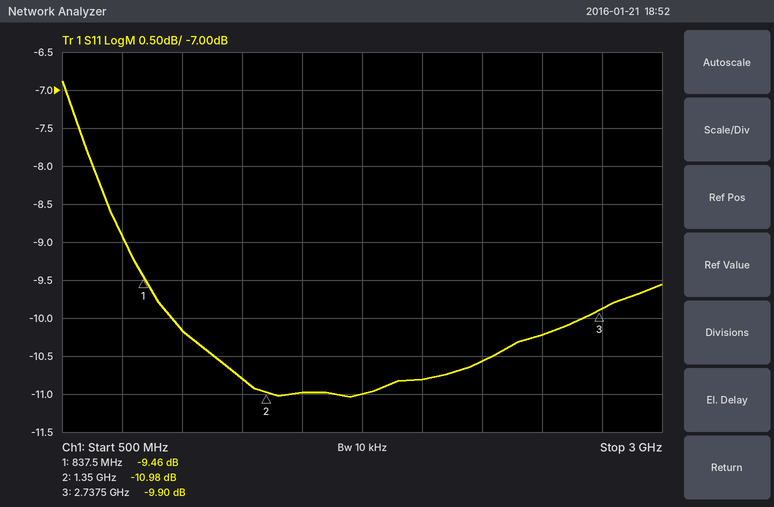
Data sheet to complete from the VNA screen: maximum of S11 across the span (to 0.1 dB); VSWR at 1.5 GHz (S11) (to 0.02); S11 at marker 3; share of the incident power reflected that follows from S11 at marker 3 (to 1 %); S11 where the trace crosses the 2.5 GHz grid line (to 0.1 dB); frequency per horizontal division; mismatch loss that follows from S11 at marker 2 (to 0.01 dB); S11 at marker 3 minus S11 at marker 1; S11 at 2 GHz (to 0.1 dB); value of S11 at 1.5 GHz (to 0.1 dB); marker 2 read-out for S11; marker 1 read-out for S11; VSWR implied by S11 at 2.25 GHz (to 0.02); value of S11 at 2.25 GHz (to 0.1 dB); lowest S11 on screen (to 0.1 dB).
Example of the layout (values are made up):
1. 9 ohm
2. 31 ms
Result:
1. -6.9 dB
2. 1.78
3. -9.90 dB
4. 10 %
5. -10.2 dB
6. 250 MHz
7. 0.36 dB
8. -0.44 dB
9. -10.8 dB
10. -11.0 dB
11. -10.98 dB
12. -9.46 dB
13. 1.84
14. -10.6 dB
15. -11.0 dB
